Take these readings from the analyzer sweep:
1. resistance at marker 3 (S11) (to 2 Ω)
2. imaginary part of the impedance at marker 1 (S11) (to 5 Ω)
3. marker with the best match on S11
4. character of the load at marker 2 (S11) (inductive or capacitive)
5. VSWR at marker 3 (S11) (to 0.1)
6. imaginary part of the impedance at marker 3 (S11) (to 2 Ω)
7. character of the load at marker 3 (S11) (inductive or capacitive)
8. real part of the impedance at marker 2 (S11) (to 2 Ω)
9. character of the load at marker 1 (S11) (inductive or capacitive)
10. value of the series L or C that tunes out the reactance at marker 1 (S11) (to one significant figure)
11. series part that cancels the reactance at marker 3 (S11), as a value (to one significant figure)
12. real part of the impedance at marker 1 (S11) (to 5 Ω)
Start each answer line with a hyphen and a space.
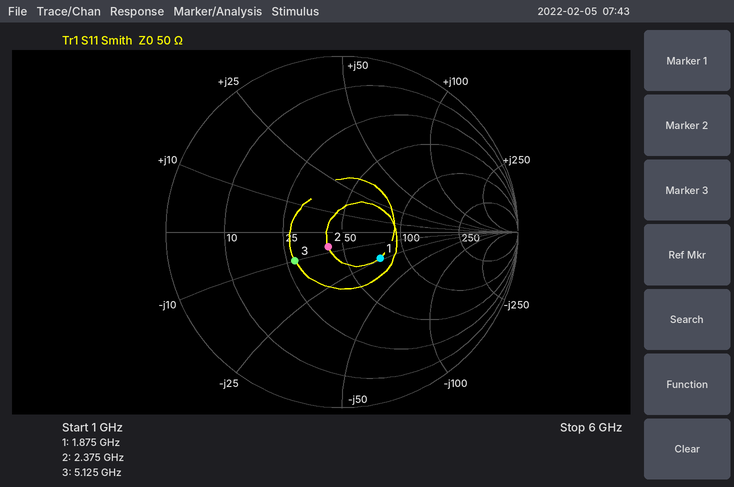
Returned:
- 28 Ω
- -25 Ω
- marker 2
- capacitive
- 1.9
- -10 Ω
- capacitive
- 42 Ω
- capacitive
- 2 nH
- 300 pH
- 75 Ω
